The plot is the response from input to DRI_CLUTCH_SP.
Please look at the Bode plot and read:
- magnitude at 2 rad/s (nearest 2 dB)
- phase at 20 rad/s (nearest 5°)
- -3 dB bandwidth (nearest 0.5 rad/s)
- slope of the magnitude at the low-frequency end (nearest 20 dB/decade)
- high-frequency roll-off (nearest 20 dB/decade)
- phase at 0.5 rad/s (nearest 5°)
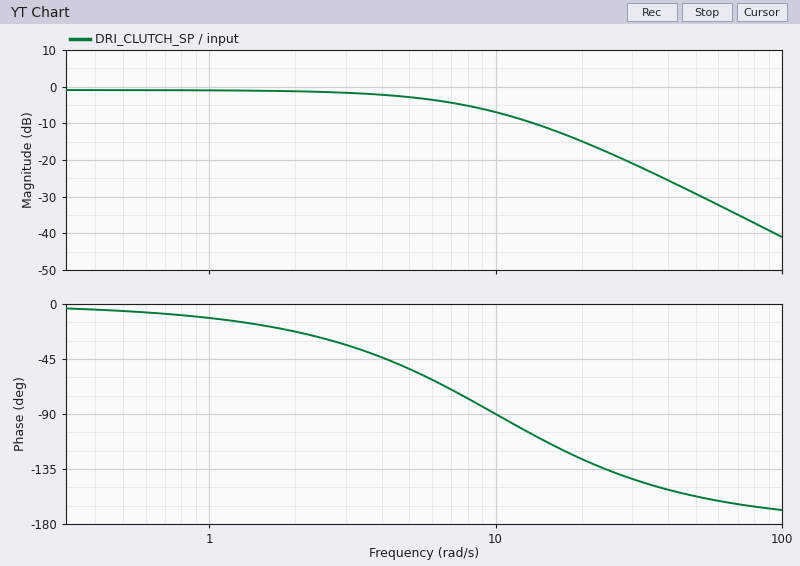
-2 dB
-125°
6.5 rad/s
0 dB/decade
-40 dB/decade
-5°
